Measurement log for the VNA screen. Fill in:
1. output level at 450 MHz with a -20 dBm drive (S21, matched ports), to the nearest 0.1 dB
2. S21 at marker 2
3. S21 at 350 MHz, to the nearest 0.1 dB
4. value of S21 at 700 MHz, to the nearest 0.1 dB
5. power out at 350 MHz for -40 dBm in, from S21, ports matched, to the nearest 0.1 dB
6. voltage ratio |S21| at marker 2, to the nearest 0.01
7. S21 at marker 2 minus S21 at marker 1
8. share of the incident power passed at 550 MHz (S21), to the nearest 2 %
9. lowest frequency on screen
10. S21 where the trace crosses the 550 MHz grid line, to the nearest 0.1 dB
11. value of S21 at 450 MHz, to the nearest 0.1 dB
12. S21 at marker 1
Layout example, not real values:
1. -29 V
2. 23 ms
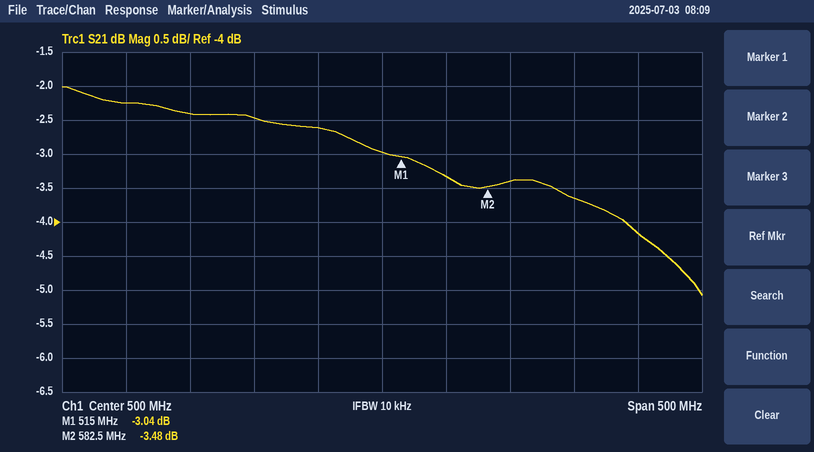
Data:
1. -22.6 dBm
2. -3.48 dB
3. -2.4 dB
4. -4.2 dB
5. -42.4 dBm
6. 0.67
7. -0.44 dB
8. 46 %
9. 250 MHz
10. -3.3 dB
11. -2.6 dB
12. -3.04 dB
